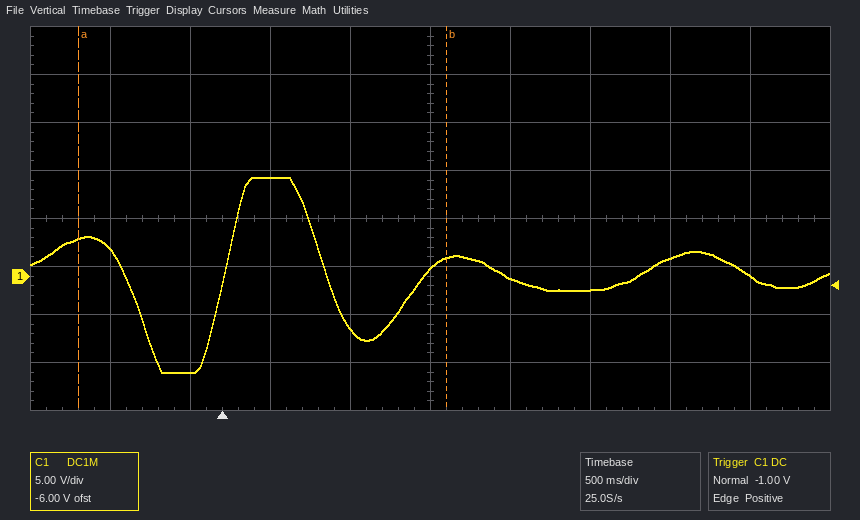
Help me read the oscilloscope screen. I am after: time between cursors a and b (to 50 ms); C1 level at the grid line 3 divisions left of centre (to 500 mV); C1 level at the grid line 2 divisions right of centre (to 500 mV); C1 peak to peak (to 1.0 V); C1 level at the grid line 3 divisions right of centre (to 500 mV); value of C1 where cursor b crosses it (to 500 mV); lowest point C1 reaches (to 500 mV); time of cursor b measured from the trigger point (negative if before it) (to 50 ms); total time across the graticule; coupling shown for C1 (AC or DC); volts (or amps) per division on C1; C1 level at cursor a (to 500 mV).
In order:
2.30 s
-10.0 V
-1.5 V
20.0 V
2.0 V
2.0 V
-10.0 V
+1.40 s
5 s
DC
5 V
4.0 V
